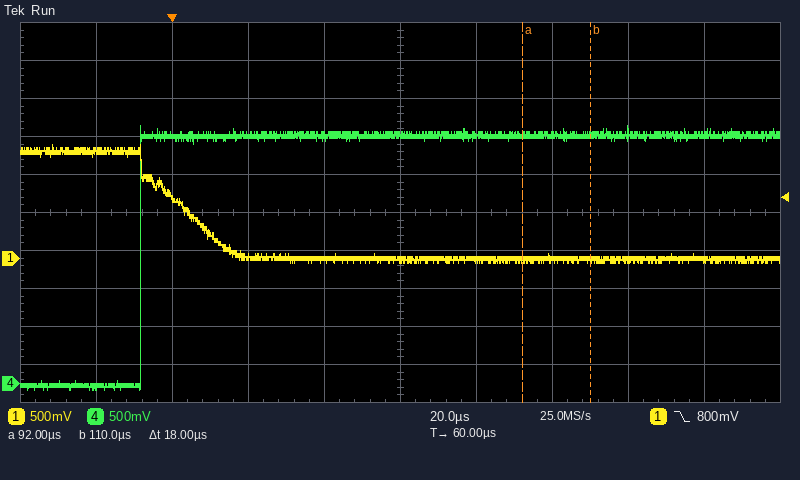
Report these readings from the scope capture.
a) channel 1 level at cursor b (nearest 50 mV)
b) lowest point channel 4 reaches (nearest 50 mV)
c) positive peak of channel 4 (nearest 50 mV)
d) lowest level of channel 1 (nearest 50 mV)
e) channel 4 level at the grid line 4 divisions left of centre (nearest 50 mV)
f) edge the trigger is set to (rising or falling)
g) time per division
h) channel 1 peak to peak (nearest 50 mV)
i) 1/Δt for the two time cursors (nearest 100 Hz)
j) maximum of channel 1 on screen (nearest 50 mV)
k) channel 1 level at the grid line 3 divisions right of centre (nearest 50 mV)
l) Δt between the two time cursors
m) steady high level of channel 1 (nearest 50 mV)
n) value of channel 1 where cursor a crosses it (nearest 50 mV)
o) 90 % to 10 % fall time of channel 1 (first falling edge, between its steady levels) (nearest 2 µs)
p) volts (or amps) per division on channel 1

0 mV
-100 mV
3.40 V
-50 mV
-50 mV
falling
20 µs
1.55 V
55.6 kHz
1.50 V
0 mV
18 µs
1.40 V
0 mV
22 µs
500 mV
